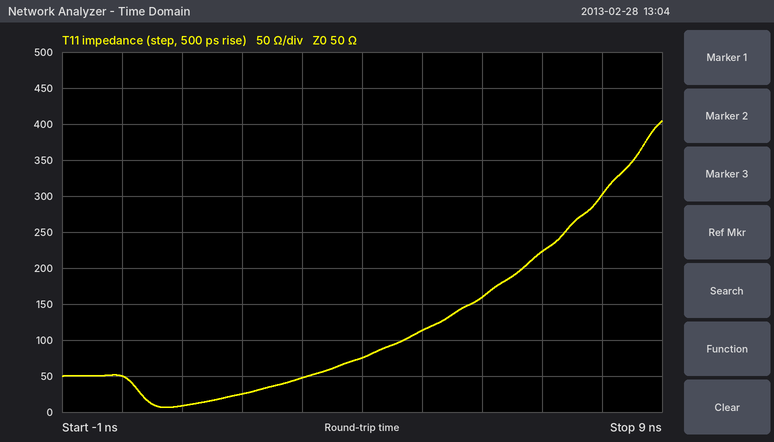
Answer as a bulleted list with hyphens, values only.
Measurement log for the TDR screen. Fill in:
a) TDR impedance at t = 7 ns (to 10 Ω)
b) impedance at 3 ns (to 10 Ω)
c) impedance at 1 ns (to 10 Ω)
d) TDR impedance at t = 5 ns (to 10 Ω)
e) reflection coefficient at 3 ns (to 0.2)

- 220 Ω
- 50 Ω
- 10 Ω
- 110 Ω
- 0.0
